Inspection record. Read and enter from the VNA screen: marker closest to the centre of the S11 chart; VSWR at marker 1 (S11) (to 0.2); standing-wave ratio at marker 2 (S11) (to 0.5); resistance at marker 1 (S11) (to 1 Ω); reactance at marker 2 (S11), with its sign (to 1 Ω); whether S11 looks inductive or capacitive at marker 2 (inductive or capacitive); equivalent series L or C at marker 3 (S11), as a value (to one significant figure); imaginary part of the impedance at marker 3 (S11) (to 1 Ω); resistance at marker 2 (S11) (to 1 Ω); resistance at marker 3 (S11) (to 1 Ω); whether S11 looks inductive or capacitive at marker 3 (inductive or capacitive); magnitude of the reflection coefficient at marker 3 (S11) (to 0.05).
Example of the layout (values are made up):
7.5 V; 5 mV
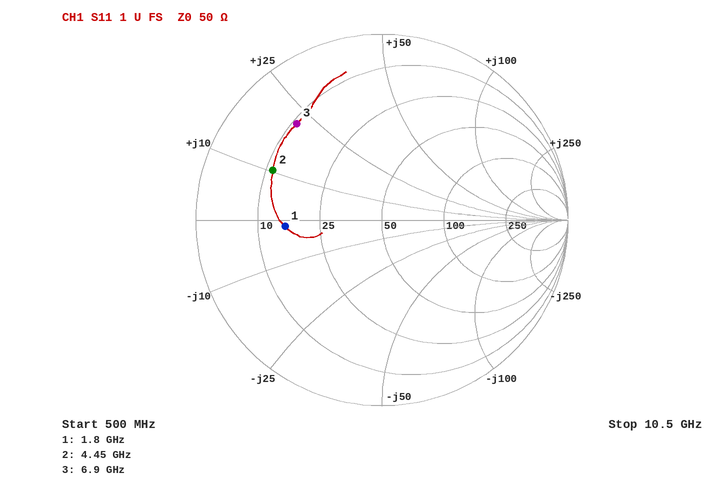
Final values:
marker 1; 3.2; 4.5; 16 Ω; +10 Ω; inductive; 500 pH; +22 Ω; 11 Ω; 11 Ω; inductive; 0.70
